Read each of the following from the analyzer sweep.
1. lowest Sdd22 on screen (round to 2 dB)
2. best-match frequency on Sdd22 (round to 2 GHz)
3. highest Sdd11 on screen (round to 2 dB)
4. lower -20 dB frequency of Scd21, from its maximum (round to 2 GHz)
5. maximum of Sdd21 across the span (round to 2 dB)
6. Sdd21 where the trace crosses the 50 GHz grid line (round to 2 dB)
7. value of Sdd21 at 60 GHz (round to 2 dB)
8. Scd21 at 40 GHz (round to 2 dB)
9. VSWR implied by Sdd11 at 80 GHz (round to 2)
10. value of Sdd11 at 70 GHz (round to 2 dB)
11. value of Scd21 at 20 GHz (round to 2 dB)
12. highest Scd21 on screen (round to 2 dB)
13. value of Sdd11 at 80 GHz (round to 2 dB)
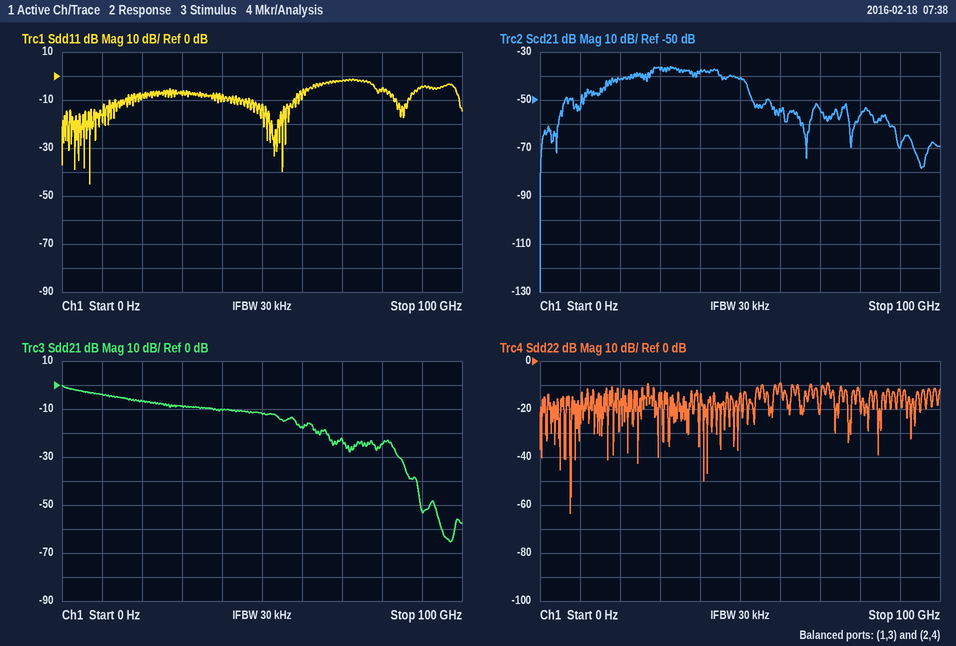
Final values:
-64 dB
8 GHz
-2 dB
6 GHz
0 dB
-12 dB
-18 dB
-38 dB
4
-2 dB
-42 dB
-36 dB
-6 dB
